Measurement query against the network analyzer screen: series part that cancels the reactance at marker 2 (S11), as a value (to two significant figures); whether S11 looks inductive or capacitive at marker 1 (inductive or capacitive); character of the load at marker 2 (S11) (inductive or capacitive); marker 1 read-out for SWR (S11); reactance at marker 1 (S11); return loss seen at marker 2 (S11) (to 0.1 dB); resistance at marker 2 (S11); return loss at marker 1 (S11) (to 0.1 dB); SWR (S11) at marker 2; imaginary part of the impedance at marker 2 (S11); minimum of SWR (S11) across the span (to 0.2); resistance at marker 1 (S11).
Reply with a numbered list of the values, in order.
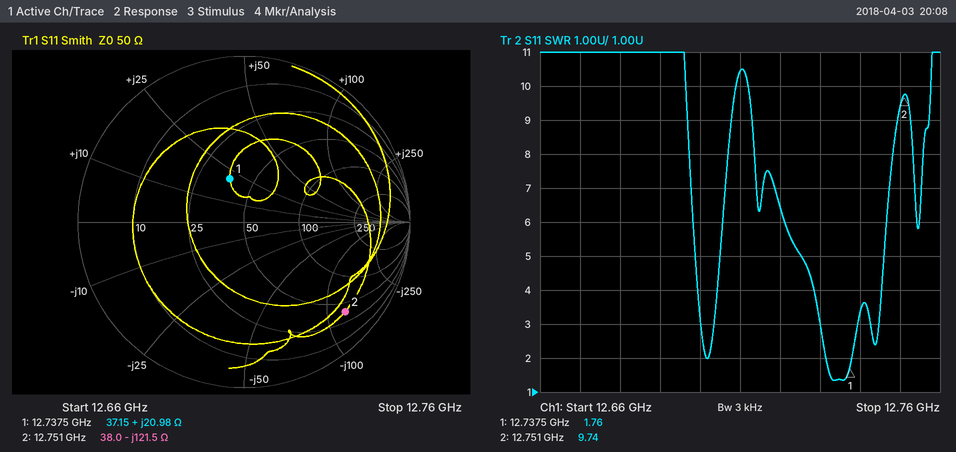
1. 1.5 nH
2. inductive
3. capacitive
4. 1.76
5. +20.98 Ω
6. 1.8 dB
7. 38.0 Ω
8. 11.2 dB
9. 9.74
10. -121.5 Ω
11. 1.4
12. 37.15 Ω
